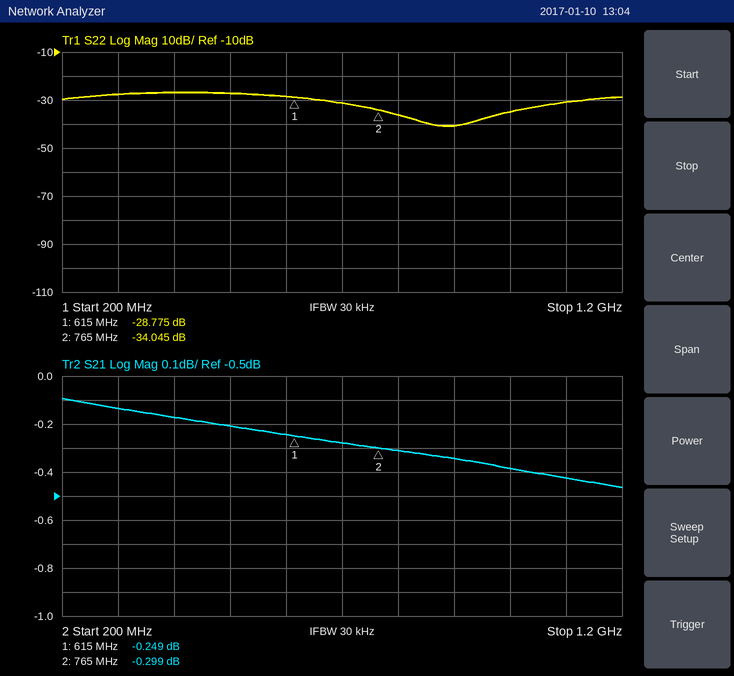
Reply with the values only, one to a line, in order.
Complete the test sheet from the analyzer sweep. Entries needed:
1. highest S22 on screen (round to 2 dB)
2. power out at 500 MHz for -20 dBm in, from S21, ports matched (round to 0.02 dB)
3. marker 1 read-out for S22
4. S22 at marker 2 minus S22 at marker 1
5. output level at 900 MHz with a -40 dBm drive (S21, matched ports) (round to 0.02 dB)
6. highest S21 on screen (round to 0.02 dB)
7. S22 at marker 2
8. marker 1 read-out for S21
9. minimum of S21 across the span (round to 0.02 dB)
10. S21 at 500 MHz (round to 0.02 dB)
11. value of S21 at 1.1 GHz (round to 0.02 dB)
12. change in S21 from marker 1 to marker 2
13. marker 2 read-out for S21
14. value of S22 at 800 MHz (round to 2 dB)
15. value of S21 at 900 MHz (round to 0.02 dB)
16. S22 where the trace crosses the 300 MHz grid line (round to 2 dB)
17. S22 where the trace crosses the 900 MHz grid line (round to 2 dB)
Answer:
-26 dB
-20.20 dBm
-28.775 dB
-5.270 dB
-40.34 dBm
-0.10 dB
-34.045 dB
-0.249 dB
-0.46 dB
-0.20 dB
-0.42 dB
-0.050 dB
-0.299 dB
-36 dB
-0.34 dB
-28 dB
-40 dB
